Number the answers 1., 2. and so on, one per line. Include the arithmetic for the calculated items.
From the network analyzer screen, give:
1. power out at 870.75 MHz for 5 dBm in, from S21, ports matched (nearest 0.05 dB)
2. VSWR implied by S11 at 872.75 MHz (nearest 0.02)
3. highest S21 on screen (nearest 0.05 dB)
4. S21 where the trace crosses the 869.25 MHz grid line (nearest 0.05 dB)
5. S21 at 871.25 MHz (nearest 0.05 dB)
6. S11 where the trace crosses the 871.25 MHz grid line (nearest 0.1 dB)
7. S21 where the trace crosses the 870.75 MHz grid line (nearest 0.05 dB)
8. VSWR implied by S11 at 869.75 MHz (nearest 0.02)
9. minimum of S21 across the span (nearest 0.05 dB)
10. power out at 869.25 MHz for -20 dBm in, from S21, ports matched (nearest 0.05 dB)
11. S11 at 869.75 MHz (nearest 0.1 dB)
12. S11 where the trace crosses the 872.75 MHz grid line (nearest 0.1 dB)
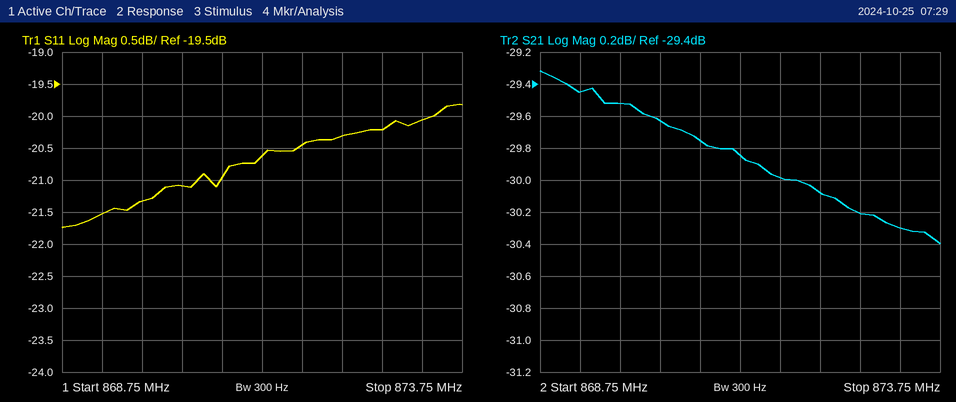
1. 5 dBm + (-29.75 dB) = -24.75 dBm
2. |Γ| = 10^(-20.2/20) = 0.0977; VSWR = (1 + 0.0977)/(1 − 0.0977) ≈ 1.22
3. -29.30 dB
4. -29.45 dB
5. -29.85 dB
6. -20.6 dB
7. -29.75 dB
8. |Γ| = 10^(-21.3/20) = 0.0861; VSWR = (1 + 0.0861)/(1 − 0.0861) ≈ 1.19, so 1.18 to the nearest 0.02
9. -30.40 dB
10. -20 dBm + (-29.45 dB) = -49.45 dBm
11. -21.3 dB
12. -20.2 dB
